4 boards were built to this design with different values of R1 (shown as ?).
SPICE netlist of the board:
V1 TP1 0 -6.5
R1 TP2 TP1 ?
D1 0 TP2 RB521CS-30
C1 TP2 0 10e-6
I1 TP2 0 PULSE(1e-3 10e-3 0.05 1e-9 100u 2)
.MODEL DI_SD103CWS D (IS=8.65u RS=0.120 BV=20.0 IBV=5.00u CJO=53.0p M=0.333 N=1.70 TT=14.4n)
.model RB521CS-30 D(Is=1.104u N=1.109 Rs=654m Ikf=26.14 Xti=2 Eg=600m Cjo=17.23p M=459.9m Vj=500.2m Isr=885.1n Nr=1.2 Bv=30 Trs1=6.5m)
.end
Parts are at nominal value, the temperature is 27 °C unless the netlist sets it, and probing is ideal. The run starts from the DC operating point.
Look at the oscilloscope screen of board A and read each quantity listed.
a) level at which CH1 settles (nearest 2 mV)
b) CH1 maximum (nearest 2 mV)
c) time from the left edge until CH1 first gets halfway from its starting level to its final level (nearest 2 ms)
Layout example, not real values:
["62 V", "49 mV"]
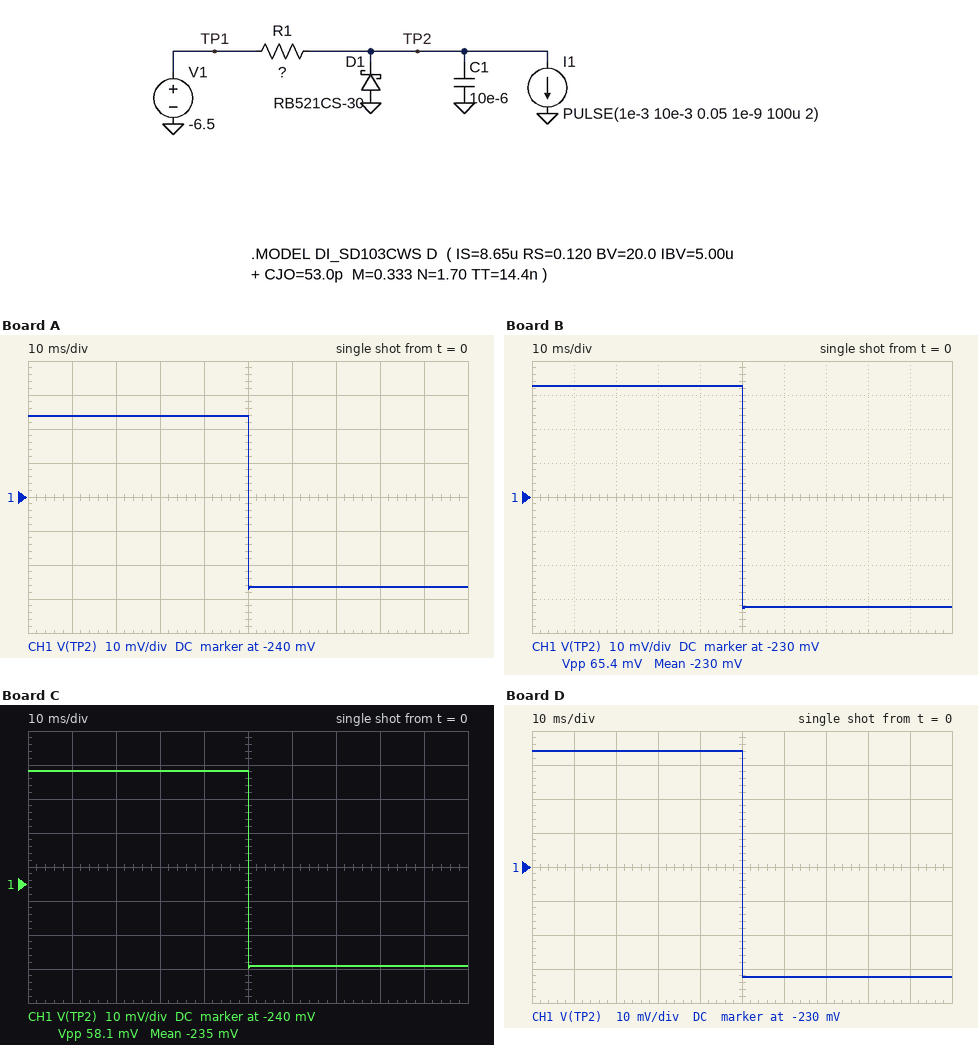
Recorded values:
["-266 mV", "-216 mV", "50 ms"]
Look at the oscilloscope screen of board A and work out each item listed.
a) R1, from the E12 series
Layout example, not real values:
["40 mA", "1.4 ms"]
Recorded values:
["3.9 kΩ"]
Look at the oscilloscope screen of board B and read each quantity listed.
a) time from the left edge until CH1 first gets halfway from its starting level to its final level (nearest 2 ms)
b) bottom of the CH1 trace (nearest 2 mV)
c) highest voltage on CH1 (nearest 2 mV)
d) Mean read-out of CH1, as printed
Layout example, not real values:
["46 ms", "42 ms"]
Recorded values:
["50 ms", "-262 mV", "-198 mV", "-230 mV"]
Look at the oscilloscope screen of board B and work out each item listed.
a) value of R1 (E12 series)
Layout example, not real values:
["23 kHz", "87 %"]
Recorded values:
["15 kΩ"]
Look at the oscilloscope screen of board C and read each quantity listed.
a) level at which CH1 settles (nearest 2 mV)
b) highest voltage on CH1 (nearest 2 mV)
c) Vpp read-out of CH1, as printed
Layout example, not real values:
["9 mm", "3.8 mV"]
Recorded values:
["-264 mV", "-206 mV", "58.1 mV"]
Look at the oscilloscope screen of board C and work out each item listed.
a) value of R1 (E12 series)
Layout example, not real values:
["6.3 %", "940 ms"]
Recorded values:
["6.8 kΩ"]
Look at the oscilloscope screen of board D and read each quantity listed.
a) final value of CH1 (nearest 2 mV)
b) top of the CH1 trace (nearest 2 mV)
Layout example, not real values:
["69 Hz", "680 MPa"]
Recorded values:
["-262 mV", "-196 mV"]
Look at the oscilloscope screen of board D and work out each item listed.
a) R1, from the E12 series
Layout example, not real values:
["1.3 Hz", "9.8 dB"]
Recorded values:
["18 kΩ"]
